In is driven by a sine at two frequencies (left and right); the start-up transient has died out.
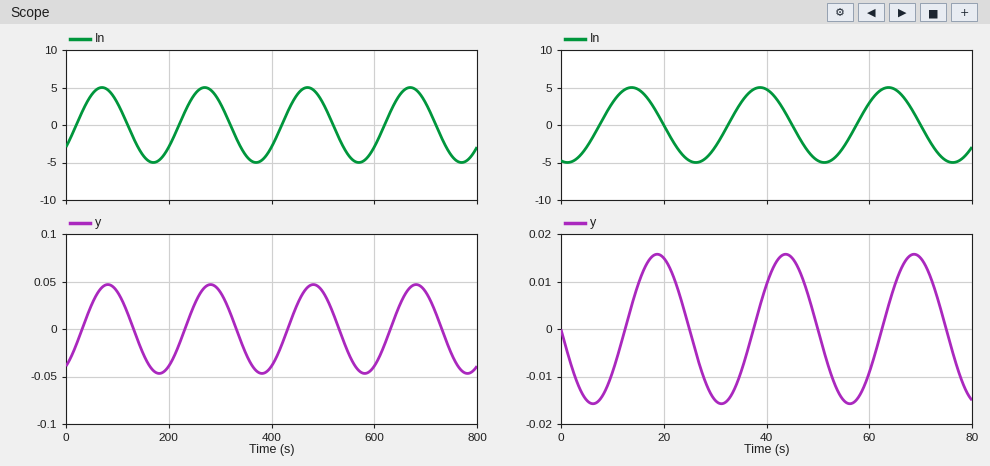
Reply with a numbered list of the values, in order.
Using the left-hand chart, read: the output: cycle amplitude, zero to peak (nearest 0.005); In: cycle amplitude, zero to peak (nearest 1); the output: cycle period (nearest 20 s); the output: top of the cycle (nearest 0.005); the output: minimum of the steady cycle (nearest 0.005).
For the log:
1. 0.045
2. 5
3. 200 s
4. 0.045
5. -0.045
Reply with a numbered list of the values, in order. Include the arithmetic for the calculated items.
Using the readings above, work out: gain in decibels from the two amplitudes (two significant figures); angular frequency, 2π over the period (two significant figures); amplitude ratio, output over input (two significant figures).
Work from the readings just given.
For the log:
1. 20 log10(0.045 / 5) = -41 dB
2. 2π / 200 = 0.031 rad/s
3. 0.045 / 5 = 0.0090
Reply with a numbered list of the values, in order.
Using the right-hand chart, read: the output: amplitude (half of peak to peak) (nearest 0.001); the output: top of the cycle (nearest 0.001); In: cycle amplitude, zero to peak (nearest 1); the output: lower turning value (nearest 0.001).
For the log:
1. 0.016
2. 0.016
3. 5
4. -0.016
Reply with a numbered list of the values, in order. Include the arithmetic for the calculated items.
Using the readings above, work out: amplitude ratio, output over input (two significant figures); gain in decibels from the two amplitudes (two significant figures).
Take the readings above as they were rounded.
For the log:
1. 0.016 / 5 = 0.0032
2. 20 log10(0.016 / 5) = -50 dB
